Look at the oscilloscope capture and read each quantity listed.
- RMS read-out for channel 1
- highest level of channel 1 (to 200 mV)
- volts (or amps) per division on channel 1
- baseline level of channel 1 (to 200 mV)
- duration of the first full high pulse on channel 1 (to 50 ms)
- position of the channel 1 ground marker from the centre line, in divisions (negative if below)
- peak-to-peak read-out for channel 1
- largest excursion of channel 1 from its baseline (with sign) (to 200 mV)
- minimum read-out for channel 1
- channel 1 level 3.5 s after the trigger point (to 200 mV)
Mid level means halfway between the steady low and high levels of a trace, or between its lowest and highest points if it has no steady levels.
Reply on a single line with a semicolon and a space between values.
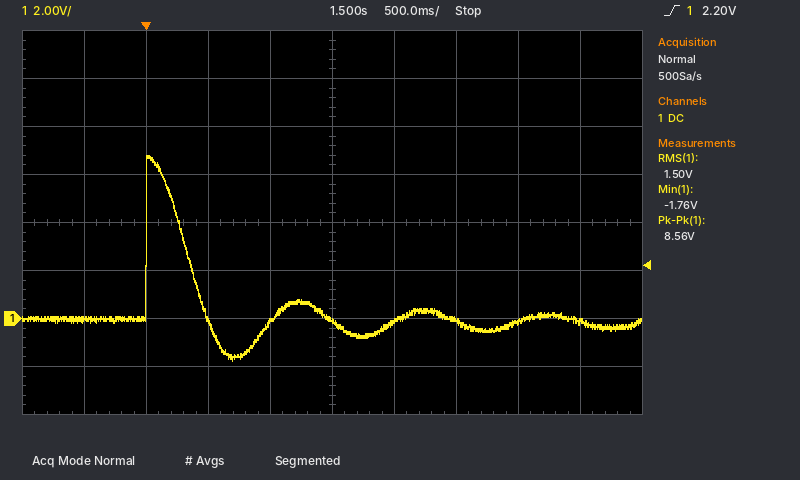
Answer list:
1.50 V; 6.8 V; 2 V; 0.0 V; 350 ms; -2.0 div; 8.56 V; +6.8 V; -1.76 V; -200 mV
